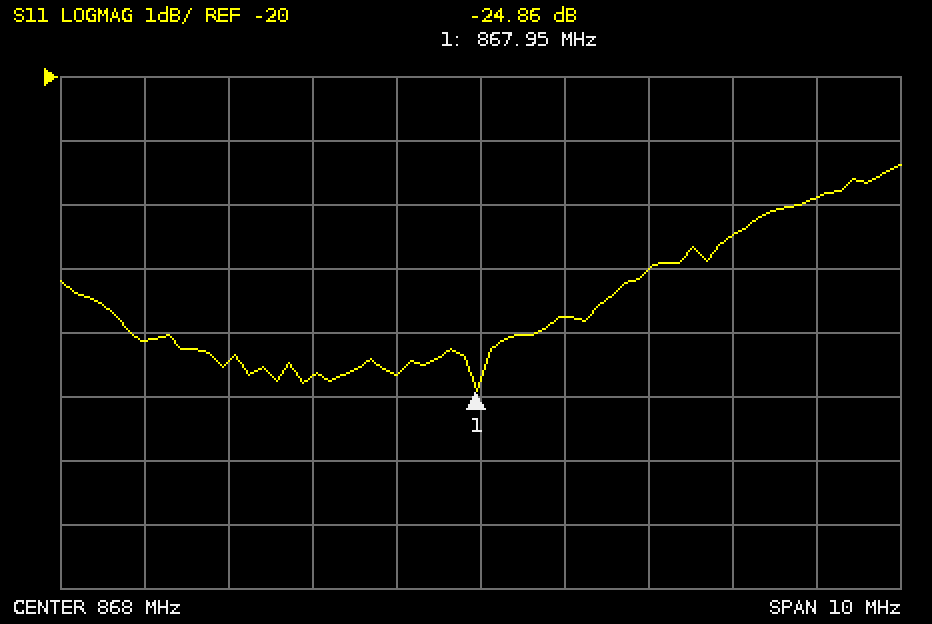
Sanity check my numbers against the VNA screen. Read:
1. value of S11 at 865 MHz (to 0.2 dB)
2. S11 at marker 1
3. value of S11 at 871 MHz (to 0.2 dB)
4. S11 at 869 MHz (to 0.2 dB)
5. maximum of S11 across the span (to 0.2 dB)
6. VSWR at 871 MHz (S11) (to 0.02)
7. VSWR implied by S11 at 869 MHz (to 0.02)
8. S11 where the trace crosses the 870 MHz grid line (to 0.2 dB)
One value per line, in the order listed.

-24.4 dB
-24.86 dB
-22.4 dB
-23.8 dB
-21.4 dB
1.16
1.14
-23.0 dB
